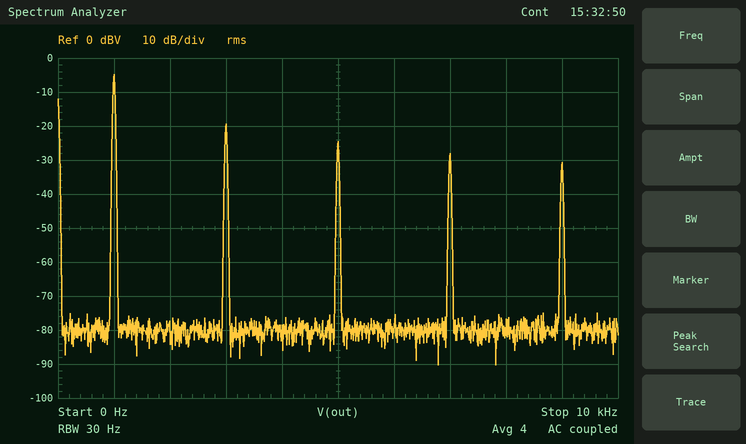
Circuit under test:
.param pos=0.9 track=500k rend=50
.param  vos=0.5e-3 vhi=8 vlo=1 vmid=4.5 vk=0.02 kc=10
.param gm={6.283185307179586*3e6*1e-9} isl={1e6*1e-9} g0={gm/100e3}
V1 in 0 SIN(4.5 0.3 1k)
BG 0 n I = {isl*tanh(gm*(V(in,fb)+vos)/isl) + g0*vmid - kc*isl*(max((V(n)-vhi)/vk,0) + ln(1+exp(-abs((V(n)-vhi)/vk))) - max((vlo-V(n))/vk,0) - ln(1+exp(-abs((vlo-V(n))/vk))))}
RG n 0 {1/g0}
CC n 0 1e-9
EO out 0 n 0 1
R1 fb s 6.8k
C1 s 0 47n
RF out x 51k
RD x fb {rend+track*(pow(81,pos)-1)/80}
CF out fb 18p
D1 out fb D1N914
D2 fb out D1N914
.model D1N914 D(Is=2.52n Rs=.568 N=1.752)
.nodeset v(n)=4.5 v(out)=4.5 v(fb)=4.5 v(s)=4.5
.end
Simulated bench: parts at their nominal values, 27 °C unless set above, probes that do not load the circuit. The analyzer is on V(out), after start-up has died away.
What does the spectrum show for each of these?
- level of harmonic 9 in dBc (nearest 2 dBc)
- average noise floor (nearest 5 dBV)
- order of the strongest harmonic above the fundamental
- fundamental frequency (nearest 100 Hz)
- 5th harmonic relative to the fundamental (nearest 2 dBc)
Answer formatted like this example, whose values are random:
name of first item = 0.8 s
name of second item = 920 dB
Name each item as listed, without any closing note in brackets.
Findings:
level of harmonic 9 in dBc = -26 dBc
average noise floor = -80 dBV
order of the strongest harmonic above the fundamental = 3
fundamental frequency = 1.0 kHz
5th harmonic relative to the fundamental = -20 dBc
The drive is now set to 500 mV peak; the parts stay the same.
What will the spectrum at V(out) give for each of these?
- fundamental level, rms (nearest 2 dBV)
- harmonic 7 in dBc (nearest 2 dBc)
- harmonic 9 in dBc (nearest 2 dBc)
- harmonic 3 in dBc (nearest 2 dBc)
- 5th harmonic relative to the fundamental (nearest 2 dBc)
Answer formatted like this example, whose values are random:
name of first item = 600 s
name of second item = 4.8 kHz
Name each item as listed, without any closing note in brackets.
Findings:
fundamental level, rms = -2 dBV
harmonic 7 in dBc = -24 dBc
harmonic 9 in dBc = -28 dBc
harmonic 3 in dBc = -16 dBc
5th harmonic relative to the fundamental = -22 dBc
